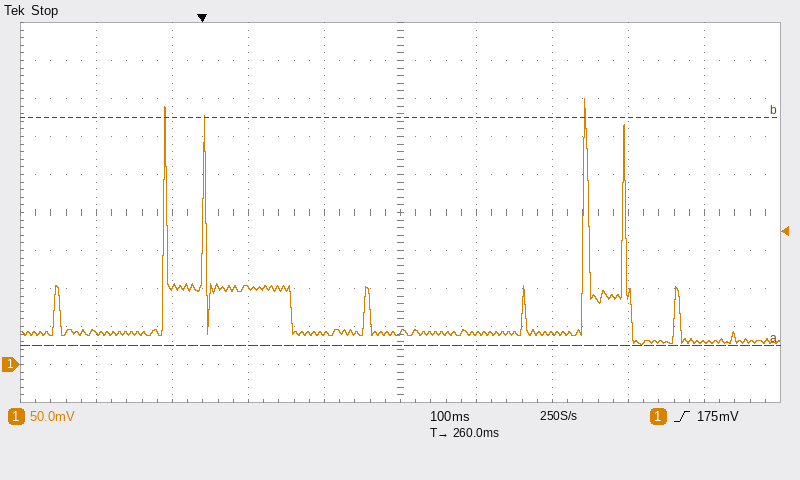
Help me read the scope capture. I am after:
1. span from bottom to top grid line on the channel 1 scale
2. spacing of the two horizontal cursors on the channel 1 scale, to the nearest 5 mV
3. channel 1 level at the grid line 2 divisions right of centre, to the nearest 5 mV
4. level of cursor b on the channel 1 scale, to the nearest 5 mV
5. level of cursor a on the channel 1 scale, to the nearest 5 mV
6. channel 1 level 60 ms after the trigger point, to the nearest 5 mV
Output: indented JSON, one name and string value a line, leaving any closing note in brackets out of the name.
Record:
{
  "span from bottom to top grid line on the channel 1 scale": "500 mV",
  "spacing of the two horizontal cursors on the channel 1 scale, to the nearest 5 mV": "300 mV",
  "channel 1 level at the grid line 2 divisions right of centre, to the nearest 5 mV": "40 mV",
  "level of cursor b on the channel 1 scale, to the nearest 5 mV": "325 mV",
  "level of cursor a on the channel 1 scale, to the nearest 5 mV": "25 mV",
  "channel 1 level 60 ms after the trigger point, to the nearest 5 mV": "100 mV"
}
